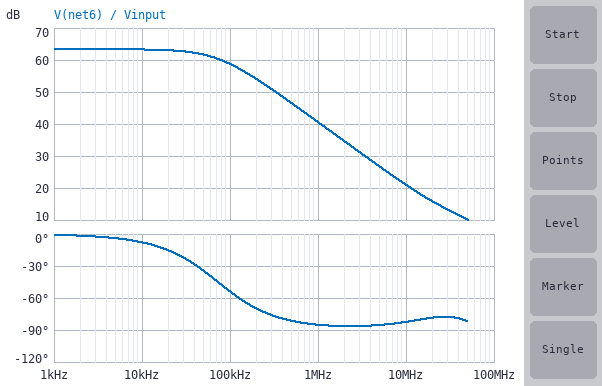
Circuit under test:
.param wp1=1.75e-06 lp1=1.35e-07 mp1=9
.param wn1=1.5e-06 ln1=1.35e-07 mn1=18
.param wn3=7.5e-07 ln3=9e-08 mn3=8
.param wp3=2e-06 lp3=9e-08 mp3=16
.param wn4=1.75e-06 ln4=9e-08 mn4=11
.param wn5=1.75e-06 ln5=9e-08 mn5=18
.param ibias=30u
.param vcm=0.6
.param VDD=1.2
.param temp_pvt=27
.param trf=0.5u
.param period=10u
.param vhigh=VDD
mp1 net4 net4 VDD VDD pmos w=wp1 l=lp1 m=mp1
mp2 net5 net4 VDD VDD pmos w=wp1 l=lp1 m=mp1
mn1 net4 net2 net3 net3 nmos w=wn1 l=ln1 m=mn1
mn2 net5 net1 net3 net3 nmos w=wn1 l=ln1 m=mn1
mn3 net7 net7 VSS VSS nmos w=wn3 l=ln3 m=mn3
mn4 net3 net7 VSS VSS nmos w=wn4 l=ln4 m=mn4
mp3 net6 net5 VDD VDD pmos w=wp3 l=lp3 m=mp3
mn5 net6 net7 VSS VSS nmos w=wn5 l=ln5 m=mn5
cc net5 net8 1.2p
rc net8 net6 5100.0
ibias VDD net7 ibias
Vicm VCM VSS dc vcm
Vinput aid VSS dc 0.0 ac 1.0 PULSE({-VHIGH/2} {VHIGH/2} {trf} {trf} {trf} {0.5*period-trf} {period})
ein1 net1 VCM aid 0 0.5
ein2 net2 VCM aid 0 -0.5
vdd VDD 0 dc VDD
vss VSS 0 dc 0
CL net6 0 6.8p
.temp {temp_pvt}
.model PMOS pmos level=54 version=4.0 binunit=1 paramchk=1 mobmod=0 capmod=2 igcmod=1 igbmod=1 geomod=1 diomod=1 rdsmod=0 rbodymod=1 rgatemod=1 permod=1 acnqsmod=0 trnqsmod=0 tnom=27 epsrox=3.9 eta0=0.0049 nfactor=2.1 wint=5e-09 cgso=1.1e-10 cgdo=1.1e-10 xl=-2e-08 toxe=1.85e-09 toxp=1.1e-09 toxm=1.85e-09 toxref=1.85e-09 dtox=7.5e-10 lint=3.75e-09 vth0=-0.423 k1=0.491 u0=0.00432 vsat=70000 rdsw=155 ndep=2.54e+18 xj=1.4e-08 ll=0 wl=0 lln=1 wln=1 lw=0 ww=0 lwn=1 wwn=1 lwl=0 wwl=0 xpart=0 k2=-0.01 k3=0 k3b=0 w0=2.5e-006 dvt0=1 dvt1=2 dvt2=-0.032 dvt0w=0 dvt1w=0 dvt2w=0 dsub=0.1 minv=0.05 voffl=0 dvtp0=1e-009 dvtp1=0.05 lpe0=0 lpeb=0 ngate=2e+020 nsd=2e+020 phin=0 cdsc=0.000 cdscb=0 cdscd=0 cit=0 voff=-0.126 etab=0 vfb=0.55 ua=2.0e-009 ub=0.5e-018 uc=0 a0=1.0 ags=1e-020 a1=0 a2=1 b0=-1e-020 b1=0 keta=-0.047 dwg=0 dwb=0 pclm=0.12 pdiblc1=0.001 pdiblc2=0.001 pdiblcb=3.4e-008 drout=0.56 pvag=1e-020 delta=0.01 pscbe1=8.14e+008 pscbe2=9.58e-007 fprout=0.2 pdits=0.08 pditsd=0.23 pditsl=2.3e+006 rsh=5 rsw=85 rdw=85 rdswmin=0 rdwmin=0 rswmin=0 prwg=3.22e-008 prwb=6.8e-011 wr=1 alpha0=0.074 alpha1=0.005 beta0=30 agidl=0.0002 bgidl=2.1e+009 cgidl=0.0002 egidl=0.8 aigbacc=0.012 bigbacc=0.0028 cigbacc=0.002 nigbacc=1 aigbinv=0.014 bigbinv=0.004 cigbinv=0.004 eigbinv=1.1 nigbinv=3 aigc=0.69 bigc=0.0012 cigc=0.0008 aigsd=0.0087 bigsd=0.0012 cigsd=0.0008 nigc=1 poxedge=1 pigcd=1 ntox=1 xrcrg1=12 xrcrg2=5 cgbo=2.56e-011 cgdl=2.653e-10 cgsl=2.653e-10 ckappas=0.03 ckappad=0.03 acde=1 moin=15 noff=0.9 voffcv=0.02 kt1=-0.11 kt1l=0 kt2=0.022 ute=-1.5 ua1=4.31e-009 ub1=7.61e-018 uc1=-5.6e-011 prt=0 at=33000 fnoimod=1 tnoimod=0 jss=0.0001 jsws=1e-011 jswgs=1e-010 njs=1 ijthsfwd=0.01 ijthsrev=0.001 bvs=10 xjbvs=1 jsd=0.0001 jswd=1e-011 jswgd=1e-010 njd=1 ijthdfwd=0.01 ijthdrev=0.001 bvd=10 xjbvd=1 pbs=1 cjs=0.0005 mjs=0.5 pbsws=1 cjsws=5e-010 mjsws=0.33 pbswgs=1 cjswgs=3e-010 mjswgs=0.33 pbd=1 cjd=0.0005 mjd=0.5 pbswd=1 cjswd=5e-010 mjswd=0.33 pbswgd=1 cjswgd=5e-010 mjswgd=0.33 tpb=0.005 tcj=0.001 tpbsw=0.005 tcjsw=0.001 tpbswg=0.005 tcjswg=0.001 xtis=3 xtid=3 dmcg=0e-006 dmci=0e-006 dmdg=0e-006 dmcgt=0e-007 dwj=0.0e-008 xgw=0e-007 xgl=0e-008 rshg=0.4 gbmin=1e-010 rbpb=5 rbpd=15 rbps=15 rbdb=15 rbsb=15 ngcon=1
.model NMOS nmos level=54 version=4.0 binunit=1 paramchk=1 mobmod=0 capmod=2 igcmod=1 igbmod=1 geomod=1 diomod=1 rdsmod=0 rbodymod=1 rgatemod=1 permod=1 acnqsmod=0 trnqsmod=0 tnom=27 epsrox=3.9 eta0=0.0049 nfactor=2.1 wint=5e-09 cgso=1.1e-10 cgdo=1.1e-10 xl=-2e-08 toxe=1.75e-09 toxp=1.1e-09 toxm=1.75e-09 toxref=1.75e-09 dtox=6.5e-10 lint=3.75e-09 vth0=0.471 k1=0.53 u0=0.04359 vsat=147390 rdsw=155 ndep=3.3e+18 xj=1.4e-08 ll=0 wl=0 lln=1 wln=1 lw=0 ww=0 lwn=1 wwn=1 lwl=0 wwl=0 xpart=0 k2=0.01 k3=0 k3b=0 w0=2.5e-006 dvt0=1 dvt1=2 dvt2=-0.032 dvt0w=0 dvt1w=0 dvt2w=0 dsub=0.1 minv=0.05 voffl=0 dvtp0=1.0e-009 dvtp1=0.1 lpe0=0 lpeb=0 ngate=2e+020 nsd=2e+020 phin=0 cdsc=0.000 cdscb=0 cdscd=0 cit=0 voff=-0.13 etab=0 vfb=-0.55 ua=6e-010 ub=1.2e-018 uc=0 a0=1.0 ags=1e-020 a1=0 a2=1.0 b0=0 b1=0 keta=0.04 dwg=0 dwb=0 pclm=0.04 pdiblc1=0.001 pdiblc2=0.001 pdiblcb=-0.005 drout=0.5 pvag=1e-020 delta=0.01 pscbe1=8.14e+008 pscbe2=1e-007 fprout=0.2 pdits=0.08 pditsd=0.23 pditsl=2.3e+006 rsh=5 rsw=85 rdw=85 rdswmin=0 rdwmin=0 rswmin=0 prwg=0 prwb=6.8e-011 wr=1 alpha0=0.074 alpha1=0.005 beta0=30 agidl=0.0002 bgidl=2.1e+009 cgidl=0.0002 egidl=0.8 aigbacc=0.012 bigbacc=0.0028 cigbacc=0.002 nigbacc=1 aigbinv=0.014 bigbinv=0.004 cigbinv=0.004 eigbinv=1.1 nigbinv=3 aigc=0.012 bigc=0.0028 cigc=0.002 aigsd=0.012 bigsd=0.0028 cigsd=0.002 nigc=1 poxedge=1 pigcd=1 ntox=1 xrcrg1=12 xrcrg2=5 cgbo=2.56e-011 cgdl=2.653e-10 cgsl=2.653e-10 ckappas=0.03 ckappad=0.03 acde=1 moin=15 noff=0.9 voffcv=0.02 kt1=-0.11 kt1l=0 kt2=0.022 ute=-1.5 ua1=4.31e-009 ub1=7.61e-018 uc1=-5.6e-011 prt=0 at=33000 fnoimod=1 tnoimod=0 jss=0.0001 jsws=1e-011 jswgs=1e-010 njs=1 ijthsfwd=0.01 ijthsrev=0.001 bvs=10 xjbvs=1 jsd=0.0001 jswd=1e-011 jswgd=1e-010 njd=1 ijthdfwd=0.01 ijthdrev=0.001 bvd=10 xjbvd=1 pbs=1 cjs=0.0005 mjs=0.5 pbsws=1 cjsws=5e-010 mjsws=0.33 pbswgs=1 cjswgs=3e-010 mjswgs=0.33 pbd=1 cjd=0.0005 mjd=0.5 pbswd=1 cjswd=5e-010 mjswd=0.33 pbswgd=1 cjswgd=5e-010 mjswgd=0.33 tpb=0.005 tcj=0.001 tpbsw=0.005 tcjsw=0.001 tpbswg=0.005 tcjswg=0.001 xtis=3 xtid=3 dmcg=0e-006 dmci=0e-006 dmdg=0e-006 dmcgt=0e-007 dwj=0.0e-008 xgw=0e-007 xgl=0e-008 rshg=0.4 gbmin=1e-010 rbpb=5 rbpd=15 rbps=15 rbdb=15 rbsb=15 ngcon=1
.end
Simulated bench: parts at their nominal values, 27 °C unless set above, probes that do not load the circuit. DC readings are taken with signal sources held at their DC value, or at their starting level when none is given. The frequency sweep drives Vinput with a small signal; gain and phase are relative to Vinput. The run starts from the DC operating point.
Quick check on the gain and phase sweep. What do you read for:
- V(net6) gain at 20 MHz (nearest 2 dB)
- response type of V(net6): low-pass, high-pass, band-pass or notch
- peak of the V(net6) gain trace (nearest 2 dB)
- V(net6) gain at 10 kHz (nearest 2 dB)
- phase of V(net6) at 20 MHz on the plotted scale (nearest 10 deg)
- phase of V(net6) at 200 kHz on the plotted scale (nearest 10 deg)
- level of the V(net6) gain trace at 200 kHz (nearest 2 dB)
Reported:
16 dB
low-pass
64 dB
64 dB
-80 deg
-70 deg
54 dB
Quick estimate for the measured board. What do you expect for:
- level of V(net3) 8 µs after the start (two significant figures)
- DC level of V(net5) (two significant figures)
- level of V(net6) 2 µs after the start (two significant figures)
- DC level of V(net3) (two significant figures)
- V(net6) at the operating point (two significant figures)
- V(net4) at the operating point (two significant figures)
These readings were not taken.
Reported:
470 mV
680 mV
1.2 V
210 mV
680 mV
680 mV
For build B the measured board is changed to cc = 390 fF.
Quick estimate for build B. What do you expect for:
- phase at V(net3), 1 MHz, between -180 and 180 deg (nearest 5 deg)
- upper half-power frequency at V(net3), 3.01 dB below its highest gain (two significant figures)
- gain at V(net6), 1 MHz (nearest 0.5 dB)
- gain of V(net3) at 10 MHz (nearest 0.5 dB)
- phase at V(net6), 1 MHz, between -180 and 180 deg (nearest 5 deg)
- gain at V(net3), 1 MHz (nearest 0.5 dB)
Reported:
145 deg
210 kHz
49.5 dB
-26.0 dB
-80 deg
-22.5 dB
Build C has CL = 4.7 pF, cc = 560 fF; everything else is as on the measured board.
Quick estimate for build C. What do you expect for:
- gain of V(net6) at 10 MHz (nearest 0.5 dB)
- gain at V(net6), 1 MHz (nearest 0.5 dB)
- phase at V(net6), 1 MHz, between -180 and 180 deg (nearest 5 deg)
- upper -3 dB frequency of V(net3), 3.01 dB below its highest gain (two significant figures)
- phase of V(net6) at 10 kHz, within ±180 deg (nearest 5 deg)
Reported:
27.0 dB
47.0 dB
-80 deg
150 kHz
-5 deg
